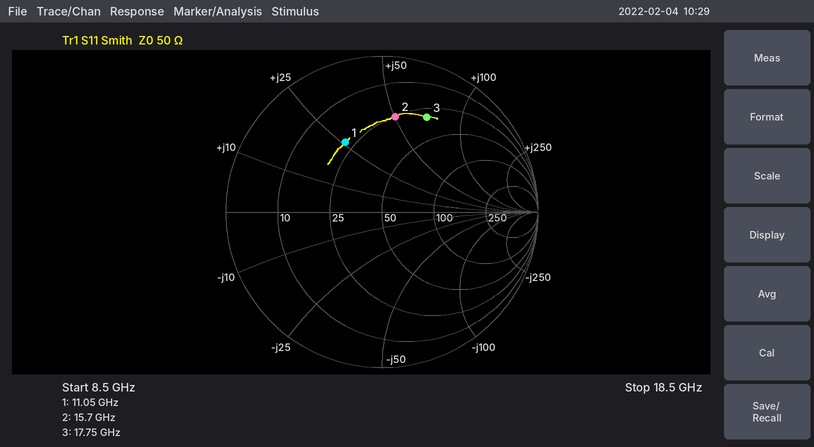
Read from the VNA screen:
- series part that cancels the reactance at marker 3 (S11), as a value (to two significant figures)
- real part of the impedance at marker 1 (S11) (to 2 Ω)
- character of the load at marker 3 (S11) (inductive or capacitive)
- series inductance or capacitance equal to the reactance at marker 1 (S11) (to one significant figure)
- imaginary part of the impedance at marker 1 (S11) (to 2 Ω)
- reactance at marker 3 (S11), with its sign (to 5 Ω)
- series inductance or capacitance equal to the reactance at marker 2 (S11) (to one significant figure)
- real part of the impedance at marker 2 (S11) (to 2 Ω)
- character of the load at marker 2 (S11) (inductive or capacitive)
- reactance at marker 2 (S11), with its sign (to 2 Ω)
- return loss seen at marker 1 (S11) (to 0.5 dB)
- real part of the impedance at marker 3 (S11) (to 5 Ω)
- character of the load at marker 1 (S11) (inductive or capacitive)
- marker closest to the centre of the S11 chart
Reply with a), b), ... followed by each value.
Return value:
a) 130 fF
b) 22 Ω
c) inductive
d) 400 pH
e) +26 Ω
f) +70 Ω
g) 500 pH
h) 26 Ω
i) inductive
j) +50 Ω
k) 6.0 dB
l) 30 Ω
m) inductive
n) marker 1
